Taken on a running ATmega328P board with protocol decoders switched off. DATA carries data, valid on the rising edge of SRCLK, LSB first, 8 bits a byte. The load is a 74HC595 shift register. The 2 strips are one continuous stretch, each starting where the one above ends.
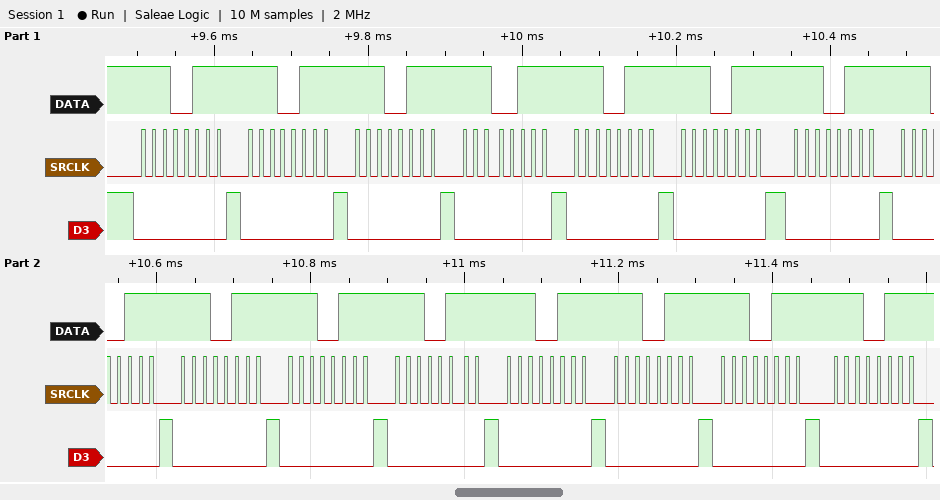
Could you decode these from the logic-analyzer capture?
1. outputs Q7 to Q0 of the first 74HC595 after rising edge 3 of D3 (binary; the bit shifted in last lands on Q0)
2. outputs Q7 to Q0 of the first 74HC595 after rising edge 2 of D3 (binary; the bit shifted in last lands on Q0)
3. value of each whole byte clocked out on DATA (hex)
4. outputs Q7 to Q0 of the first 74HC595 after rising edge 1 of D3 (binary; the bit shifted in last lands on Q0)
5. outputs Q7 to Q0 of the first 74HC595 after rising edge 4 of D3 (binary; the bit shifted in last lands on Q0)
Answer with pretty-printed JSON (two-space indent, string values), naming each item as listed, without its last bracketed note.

{
  "outputs Q7 to Q0 of the first 74HC595 after rising edge 3 of D3": "11100111",
  "outputs Q7 to Q0 of the first 74HC595 after rising edge 2 of D3": "11100111",
  "value of each whole byte clocked out on DATA": "0xE7 0xE7 0xE7 0xE7 0xE7 0xE7 0xE7 0xE7 0xE7 0xE7 0xE7 0xE7 0xE7 0xE7 0xE7",
  "outputs Q7 to Q0 of the first 74HC595 after rising edge 1 of D3": "11100111",
  "outputs Q7 to Q0 of the first 74HC595 after rising edge 4 of D3": "11100111"
}
